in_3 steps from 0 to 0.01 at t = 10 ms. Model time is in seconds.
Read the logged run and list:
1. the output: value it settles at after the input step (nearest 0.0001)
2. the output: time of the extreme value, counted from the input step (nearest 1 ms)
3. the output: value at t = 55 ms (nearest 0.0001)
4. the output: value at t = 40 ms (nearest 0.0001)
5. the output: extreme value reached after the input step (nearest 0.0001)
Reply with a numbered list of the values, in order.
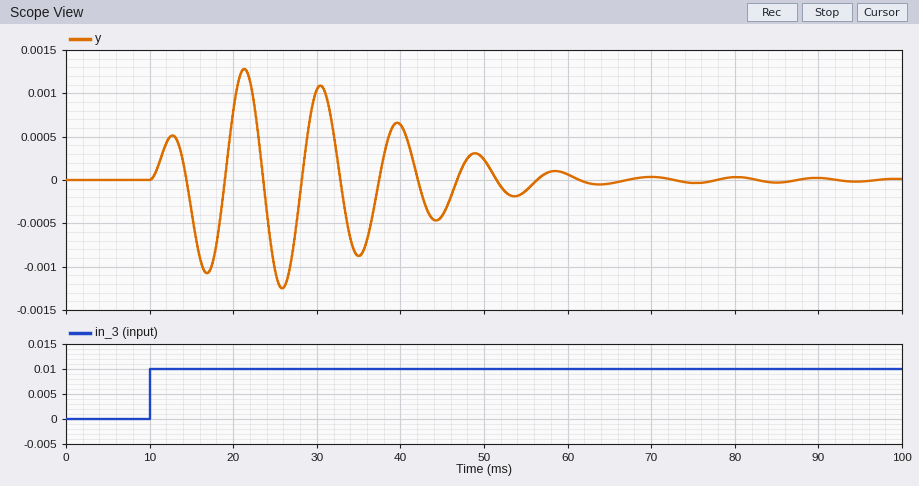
1. 0.0000
2. 11 ms
3. -0.0001
4. 0.0006
5. 0.0013
